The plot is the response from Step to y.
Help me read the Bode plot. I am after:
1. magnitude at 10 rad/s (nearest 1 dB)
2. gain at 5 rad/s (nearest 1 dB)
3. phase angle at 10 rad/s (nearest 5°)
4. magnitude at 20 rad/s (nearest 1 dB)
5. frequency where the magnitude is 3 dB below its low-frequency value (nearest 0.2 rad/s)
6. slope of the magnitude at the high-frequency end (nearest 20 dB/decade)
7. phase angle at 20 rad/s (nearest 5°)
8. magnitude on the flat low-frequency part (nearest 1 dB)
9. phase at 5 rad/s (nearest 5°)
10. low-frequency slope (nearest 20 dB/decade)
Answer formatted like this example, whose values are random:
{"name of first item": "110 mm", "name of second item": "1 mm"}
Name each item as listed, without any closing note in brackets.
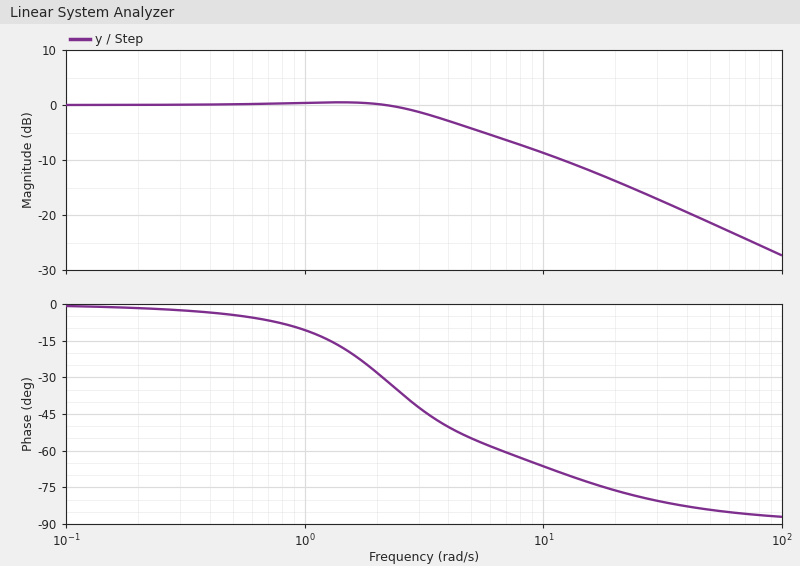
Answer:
{"magnitude at 10 rad/s": "-9 dB", "gain at 5 rad/s": "-4 dB", "phase angle at 10 rad/s": "-65°", "magnitude at 20 rad/s": "-14 dB", "frequency where the magnitude is 3 dB below its low-frequency value": "4.0 rad/s", "slope of the magnitude at the high-frequency end": "-20 dB/decade", "phase angle at 20 rad/s": "-75°", "magnitude on the flat low-frequency part": "0 dB", "phase at 5 rad/s": "-55°", "low-frequency slope": "0 dB/decade"}
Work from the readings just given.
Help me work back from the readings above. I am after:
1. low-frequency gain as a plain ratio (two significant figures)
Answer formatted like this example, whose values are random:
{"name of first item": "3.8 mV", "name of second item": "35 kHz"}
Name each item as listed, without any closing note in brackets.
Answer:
{"low-frequency gain as a plain ratio": "1.0"}
